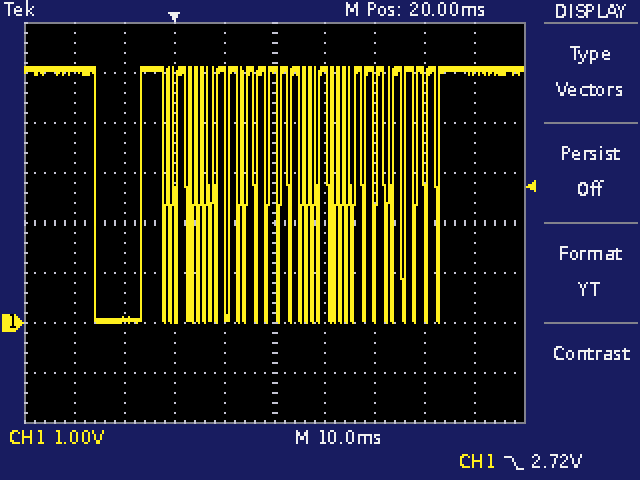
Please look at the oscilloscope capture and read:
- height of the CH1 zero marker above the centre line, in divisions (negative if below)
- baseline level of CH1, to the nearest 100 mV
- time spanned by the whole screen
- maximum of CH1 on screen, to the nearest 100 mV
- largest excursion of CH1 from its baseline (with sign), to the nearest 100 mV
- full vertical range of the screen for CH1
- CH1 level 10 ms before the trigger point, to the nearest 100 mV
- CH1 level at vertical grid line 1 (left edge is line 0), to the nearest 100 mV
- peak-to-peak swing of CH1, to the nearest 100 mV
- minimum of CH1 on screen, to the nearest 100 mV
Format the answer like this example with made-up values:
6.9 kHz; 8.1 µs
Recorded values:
-2.0 div; 5.1 V; 100 ms; 5.1 V; -5.1 V; 8 V; 100 mV; 5.1 V; 5.1 V; 0.0 V
